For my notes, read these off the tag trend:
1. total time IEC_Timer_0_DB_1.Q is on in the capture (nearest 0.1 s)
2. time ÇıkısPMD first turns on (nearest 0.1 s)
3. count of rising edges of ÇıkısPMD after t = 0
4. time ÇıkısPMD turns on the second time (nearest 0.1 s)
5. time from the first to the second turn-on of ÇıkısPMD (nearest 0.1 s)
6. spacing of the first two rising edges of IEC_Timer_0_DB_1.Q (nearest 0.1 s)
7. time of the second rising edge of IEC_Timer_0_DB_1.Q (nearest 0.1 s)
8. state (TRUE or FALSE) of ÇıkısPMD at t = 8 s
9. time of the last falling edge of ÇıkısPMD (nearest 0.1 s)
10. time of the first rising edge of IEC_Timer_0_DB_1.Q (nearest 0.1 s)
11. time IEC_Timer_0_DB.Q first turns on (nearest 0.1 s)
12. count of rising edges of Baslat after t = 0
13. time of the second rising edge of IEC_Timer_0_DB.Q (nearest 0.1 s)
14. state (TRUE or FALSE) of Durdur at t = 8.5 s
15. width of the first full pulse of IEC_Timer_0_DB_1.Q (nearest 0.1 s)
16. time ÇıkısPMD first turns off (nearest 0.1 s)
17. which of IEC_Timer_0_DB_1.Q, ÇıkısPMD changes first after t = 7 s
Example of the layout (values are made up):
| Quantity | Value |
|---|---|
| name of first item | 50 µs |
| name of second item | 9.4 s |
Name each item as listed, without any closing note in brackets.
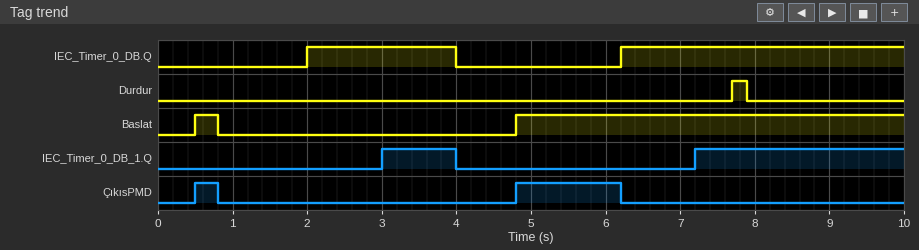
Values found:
| Quantity | Value |
|---|---|
| total time IEC_Timer_0_DB_1.Q is on in the capture | 3.8 s |
| time ÇıkısPMD first turns on | 0.5 s |
| count of rising edges of ÇıkısPMD after t = 0 | 2 |
| time ÇıkısPMD turns on the second time | 4.8 s |
| time from the first to the second turn-on of ÇıkısPMD | 4.3 s |
| spacing of the first two rising edges of IEC_Timer_0_DB_1.Q | 4.2 s |
| time of the second rising edge of IEC_Timer_0_DB_1.Q | 7.2 s |
| state (TRUE or FALSE) of ÇıkısPMD at t = 8 s | FALSE |
| time of the last falling edge of ÇıkısPMD | 6.2 s |
| time of the first rising edge of IEC_Timer_0_DB_1.Q | 3.0 s |
| time IEC_Timer_0_DB.Q first turns on | 2.0 s |
| count of rising edges of Baslat after t = 0 | 2 |
| time of the second rising edge of IEC_Timer_0_DB.Q | 6.2 s |
| state (TRUE or FALSE) of Durdur at t = 8.5 s | FALSE |
| width of the first full pulse of IEC_Timer_0_DB_1.Q | 1.0 s |
| time ÇıkısPMD first turns off | 0.8 s |
| which of IEC_Timer_0_DB_1.Q, ÇıkısPMD changes first after t = 7 s | IEC_Timer_0_DB_1.Q |
